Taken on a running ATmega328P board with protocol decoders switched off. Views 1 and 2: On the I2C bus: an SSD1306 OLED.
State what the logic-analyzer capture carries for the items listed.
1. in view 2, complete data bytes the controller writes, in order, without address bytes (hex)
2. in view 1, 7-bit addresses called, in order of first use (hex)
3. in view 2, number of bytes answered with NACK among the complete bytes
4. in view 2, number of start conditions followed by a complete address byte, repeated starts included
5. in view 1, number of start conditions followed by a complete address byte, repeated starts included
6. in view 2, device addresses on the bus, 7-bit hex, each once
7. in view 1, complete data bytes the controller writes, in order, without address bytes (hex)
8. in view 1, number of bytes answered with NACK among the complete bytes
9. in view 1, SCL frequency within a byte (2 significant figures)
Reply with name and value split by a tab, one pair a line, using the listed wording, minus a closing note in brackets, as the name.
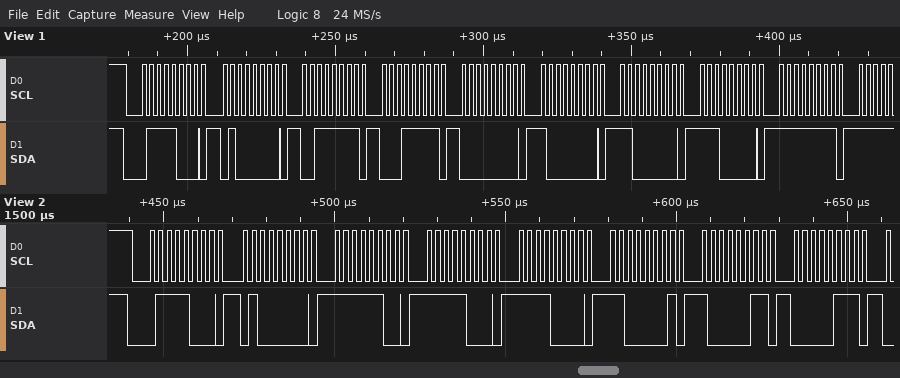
in view 2, complete data bytes the controller writes, in order, without address bytes	40 FC F8 F0 C1 83 07
in view 1, 7-bit addresses called, in order of first use	0x3C
in view 2, number of bytes answered with NACK among the complete bytes	0
in view 2, number of start conditions followed by a complete address byte, repeated starts included	1
in view 1, number of start conditions followed by a complete address byte, repeated starts included	1
in view 2, device addresses on the bus, 7-bit hex, each once	0x3C
in view 1, complete data bytes the controller writes, in order, without address bytes	40 3F 1F 00 80 C0 E0 FF
in view 1, number of bytes answered with NACK among the complete bytes	0
in view 1, SCL frequency within a byte	400 kHz
